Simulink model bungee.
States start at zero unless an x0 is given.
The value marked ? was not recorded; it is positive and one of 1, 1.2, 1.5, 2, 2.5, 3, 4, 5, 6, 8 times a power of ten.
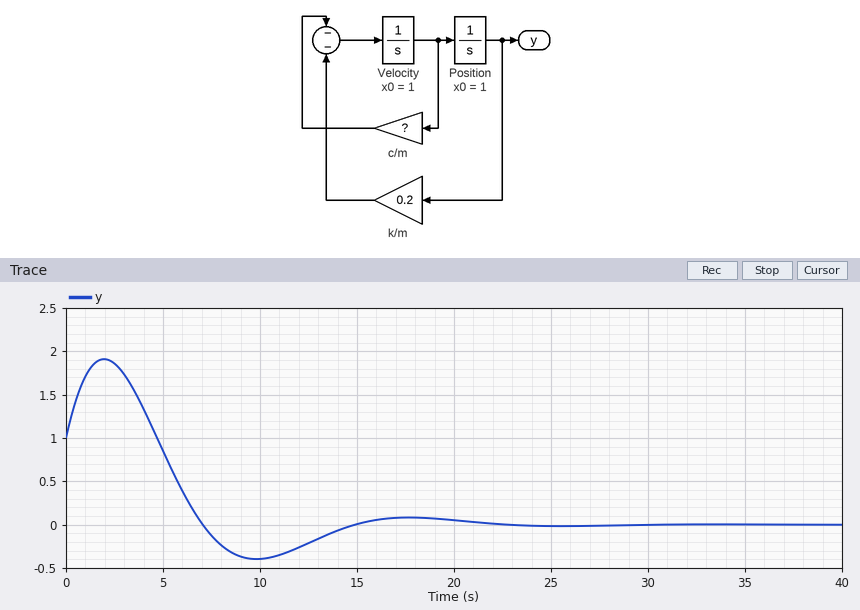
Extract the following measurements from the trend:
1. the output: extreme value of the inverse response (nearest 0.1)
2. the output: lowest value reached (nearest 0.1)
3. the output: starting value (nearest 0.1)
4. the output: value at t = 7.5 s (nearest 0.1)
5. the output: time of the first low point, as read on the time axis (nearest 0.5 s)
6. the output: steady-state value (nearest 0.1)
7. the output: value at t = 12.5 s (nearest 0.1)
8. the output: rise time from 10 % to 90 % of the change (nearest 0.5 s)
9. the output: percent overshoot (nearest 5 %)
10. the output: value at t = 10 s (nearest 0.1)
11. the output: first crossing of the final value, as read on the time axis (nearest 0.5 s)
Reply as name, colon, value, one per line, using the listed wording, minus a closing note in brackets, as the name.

the output: extreme value of the inverse response: 1.9
the output: lowest value reached: -0.4
the output: starting value: 1.0
the output: value at t = 7.5 s: -0.1
the output: time of the first low point, as read on the time axis: 10.0 s
the output: steady-state value: 0.0
the output: value at t = 12.5 s: -0.2
the output: rise time from 10 % to 90 % of the change: 2.0 s
the output: percent overshoot: 40 %
the output: value at t = 10 s: -0.4
the output: first crossing of the final value, as read on the time axis: 7.0 s
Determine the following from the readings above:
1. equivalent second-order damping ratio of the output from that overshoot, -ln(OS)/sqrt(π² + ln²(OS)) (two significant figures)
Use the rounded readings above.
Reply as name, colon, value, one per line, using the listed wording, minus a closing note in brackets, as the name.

equivalent second-order damping ratio of the output from that overshoot, -ln(OS)/sqrt(π² + ln²(OS)): 0.28
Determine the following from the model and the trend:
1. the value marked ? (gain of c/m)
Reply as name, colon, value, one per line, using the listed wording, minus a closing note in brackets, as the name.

the value marked ?: 0.4
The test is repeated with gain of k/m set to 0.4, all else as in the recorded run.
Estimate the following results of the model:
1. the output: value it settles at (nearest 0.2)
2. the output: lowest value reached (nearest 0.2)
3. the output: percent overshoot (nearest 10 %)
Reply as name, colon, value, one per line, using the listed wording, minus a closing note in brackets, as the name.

the output: value it settles at: 0.0
the output: lowest value reached: -0.6
the output: percent overshoot: 60 %
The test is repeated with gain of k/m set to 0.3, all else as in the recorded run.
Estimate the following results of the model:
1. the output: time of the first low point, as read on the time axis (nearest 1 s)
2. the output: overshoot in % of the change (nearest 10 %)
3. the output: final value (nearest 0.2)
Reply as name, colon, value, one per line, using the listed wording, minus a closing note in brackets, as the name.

the output: time of the first low point, as read on the time axis: 8 s
the output: overshoot in % of the change: 50 %
the output: final value: 0.0
